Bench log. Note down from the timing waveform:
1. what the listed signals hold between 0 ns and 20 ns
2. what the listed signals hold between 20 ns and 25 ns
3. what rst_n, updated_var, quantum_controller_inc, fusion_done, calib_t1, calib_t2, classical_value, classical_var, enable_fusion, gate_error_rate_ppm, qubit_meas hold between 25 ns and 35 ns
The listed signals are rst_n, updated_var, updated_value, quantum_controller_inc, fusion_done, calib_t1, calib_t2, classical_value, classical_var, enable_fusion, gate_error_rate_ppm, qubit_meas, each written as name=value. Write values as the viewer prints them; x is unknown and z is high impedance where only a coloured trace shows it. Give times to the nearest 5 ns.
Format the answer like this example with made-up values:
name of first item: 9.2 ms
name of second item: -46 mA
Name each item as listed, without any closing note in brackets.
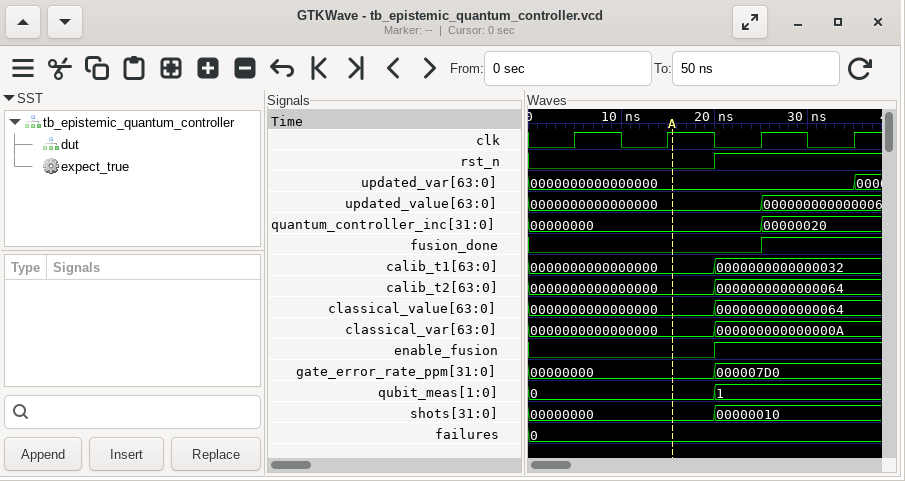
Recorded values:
what the listed signals hold between 0 ns and 20 ns: rst_n=0, updated_var=0000000000000000, updated_value=0000000000000000, quantum_controller_inc=00000000, fusion_done=0, calib_t1=0000000000000000, calib_t2=0000000000000000, classical_value=0000000000000000, classical_var=0000000000000000, enable_fusion=0, gate_error_rate_ppm=00000000, qubit_meas=0
what the listed signals hold between 20 ns and 25 ns: rst_n=1, updated_var=0000000000000000, updated_value=0000000000000000, quantum_controller_inc=00000000, fusion_done=0, calib_t1=0000000000000032, calib_t2=0000000000000064, classical_value=0000000000000064, classical_var=000000000000000A, enable_fusion=1, gate_error_rate_ppm=000007D0, qubit_meas=1
what rst_n, updated_var, quantum_controller_inc, fusion_done, calib_t1, calib_t2, classical_value, classical_var, enable_fusion, gate_error_rate_ppm, qubit_meas hold between 25 ns and 35 ns: rst_n=1, updated_var=0000000000000000, quantum_controller_inc=00000020, fusion_done=1, calib_t1=0000000000000032, calib_t2=0000000000000064, classical_value=0000000000000064, classical_var=000000000000000A, enable_fusion=1, gate_error_rate_ppm=000007D0, qubit_meas=1
